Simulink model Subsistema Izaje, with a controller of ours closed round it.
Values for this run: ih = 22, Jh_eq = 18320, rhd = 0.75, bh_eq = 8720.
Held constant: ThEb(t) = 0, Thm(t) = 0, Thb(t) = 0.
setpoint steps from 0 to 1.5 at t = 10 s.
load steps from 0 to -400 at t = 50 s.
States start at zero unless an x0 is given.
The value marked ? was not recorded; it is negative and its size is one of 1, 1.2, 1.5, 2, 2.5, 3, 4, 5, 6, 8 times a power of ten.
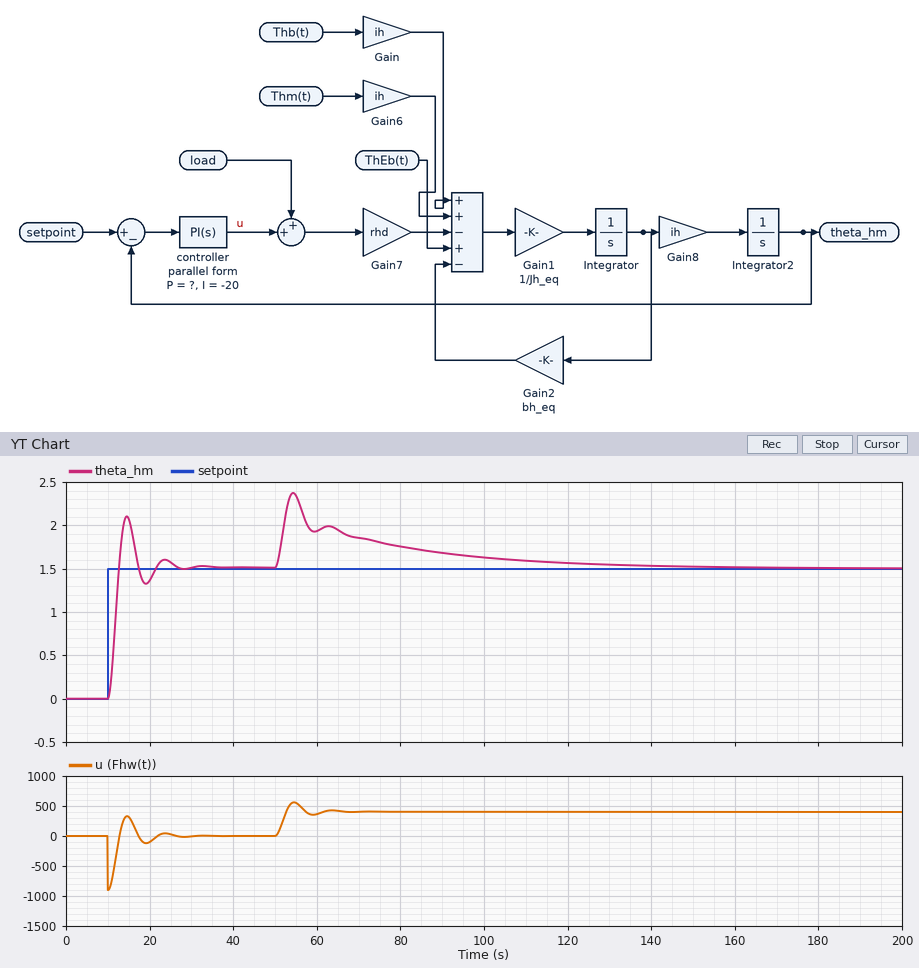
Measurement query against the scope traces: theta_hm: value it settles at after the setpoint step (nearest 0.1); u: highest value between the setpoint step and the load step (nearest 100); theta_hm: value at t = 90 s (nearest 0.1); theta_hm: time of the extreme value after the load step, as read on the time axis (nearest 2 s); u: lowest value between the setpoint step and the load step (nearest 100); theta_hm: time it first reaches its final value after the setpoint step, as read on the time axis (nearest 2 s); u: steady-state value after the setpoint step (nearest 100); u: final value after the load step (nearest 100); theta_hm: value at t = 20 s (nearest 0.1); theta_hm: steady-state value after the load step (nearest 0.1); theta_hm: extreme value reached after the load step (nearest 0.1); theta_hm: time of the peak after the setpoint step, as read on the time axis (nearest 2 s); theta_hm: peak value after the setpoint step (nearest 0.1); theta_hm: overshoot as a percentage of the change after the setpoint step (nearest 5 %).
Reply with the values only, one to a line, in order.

1.5
300
1.7
54 s
-900
12 s
0
400
1.4
1.5
2.4
14 s
2.1
40 %
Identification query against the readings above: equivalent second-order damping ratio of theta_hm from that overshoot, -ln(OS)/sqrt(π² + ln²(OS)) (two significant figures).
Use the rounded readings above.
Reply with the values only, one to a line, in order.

0.28
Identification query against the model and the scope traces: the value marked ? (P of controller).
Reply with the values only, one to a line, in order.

-600
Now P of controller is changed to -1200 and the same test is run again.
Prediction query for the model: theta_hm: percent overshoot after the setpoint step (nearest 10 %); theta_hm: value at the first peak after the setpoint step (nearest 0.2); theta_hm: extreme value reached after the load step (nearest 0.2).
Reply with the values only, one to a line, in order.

50 %
2.2
2.0
